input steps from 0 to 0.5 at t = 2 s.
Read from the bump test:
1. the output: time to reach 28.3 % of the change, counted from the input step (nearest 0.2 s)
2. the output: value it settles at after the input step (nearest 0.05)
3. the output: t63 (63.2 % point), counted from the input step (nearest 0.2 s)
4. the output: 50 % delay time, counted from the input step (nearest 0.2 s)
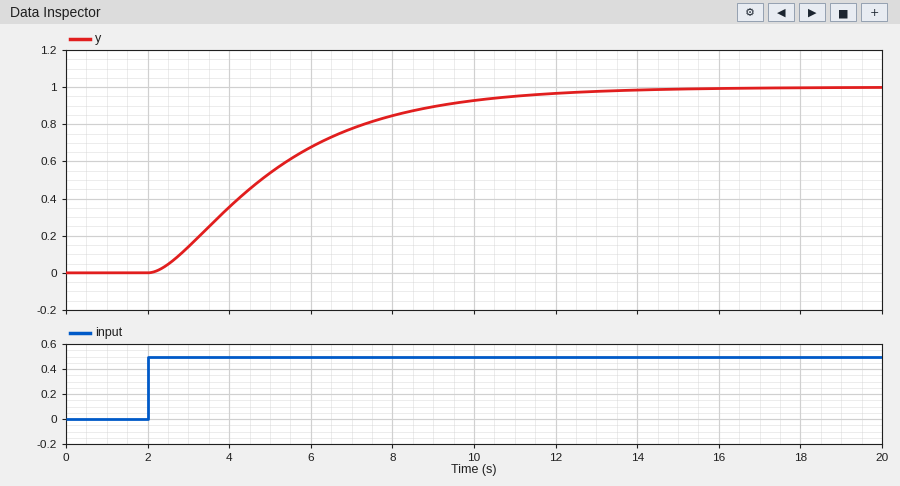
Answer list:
1.6 s
1.00
3.6 s
2.8 s
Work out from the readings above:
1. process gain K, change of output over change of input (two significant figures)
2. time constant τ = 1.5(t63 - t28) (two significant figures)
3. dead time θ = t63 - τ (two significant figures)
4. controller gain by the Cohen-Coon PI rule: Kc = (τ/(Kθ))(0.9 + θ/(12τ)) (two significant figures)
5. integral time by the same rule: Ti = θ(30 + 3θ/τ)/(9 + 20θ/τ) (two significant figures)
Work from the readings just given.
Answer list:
2.0
3.0 s
0.60 s
2.3
1.4 s
